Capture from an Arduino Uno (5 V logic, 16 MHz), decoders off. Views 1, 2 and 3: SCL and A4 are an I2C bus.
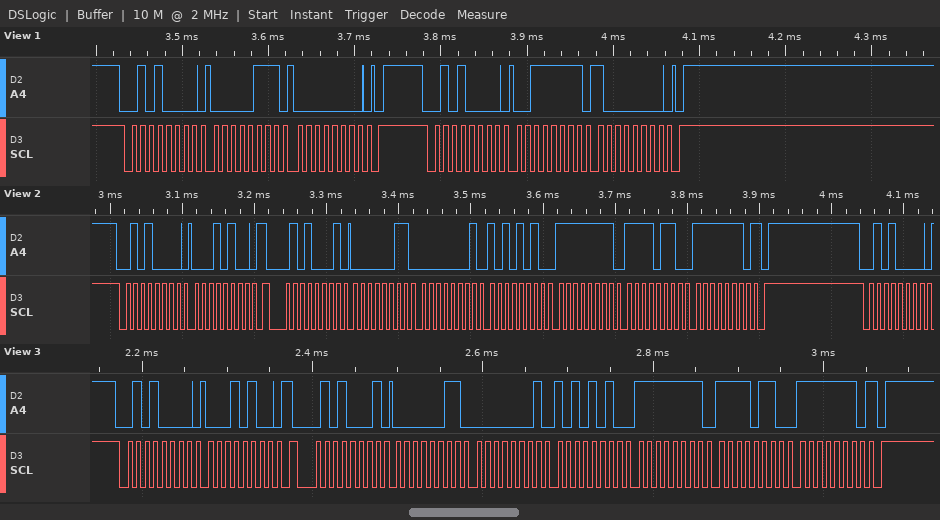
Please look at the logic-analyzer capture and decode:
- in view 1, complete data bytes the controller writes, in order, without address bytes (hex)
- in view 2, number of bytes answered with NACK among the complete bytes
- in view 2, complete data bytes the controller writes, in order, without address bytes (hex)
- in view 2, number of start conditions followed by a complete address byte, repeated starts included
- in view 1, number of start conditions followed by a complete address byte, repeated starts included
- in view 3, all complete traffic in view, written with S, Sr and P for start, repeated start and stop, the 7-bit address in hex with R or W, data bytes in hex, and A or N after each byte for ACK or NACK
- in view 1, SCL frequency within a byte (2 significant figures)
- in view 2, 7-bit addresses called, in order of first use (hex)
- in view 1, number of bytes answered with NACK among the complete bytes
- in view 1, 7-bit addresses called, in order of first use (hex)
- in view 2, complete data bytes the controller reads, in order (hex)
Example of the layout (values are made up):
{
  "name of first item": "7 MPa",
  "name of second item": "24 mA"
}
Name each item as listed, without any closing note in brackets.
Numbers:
{
  "in view 1, complete data bytes the controller writes, in order, without address bytes": "07 00 3F 80",
  "in view 2, number of bytes answered with NACK among the complete bytes": "1",
  "in view 2, complete data bytes the controller writes, in order, without address bytes": "14",
  "in view 2, number of start conditions followed by a complete address byte, repeated starts included": "3",
  "in view 1, number of start conditions followed by a complete address byte, repeated starts included": "2",
  "in view 3, all complete traffic in view, written with S, Sr and P for start, repeated start and stop, the 7-bit address in hex with R or W, data bytes in hex, and A or N after each byte for ACK or NACK": "S 28W A 14 A Sr 28R A 03 A 01 A AA A FF A F6 A FE N P",
  "in view 1, SCL frequency within a byte": "100 kHz",
  "in view 2, 7-bit addresses called, in order of first use": "0x28",
  "in view 1, number of bytes answered with NACK among the complete bytes": "0",
  "in view 1, 7-bit addresses called, in order of first use": "0x28",
  "in view 2, complete data bytes the controller reads, in order": "03 01 AA FF F6 FE"
}
